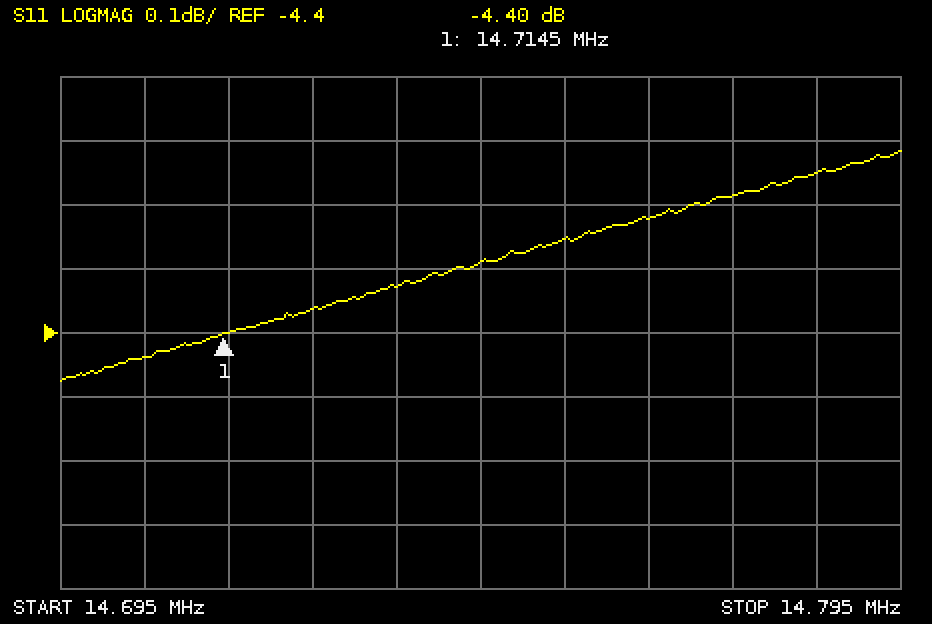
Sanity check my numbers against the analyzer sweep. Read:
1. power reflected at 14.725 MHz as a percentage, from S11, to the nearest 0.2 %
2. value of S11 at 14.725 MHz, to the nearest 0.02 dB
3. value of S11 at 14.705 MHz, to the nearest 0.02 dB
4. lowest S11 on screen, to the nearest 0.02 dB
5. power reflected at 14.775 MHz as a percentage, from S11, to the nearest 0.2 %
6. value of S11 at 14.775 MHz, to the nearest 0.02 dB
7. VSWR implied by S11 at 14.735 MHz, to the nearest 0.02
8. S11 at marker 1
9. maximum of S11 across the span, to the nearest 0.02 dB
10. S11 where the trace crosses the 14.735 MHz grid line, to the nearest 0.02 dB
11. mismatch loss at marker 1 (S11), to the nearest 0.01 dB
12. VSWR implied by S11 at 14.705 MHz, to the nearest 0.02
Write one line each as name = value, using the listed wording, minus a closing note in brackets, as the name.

power reflected at 14.725 MHz as a percentage, from S11, to the nearest 0.2 % = 36.6 %
value of S11 at 14.725 MHz, to the nearest 0.02 dB = -4.36 dB
value of S11 at 14.705 MHz, to the nearest 0.02 dB = -4.44 dB
lowest S11 on screen, to the nearest 0.02 dB = -4.48 dB
power reflected at 14.775 MHz as a percentage, from S11, to the nearest 0.2 % = 38.2 %
value of S11 at 14.775 MHz, to the nearest 0.02 dB = -4.18 dB
VSWR implied by S11 at 14.735 MHz, to the nearest 0.02 = 4.10
S11 at marker 1 = -4.40 dB
maximum of S11 across the span, to the nearest 0.02 dB = -4.12 dB
S11 where the trace crosses the 14.735 MHz grid line, to the nearest 0.02 dB = -4.32 dB
mismatch loss at marker 1 (S11), to the nearest 0.01 dB = 1.96 dB
VSWR implied by S11 at 14.705 MHz, to the nearest 0.02 = 4.00
